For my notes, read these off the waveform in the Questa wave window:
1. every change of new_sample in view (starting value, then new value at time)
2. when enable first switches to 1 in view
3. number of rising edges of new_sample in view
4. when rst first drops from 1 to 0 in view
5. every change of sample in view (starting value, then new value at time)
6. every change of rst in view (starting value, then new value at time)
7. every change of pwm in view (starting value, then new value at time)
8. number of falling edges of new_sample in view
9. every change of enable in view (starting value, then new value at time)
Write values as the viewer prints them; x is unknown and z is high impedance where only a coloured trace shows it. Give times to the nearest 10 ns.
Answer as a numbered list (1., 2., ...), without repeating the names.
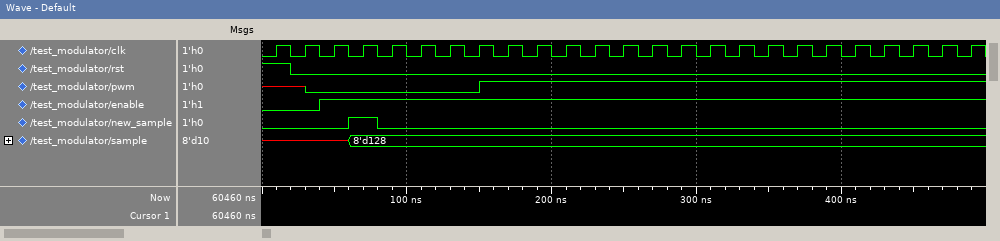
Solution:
1. 0, 1 at 60 ns, 0 at 80 ns
2. 40 ns
3. 1
4. 20 ns
5. x, 8'd128 at 60 ns
6. 1, 0 at 20 ns
7. x, 0 at 30 ns, 1 at 150 ns
8. 1
9. 0, 1 at 40 ns
